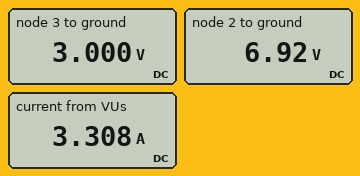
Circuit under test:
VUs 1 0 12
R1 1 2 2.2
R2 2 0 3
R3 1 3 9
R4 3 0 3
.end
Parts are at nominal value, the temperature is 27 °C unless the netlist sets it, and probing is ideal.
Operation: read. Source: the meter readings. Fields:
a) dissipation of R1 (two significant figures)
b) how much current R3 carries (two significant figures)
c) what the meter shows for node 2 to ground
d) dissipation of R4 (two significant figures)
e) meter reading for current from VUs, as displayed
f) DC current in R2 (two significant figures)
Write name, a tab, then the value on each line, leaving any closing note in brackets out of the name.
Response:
dissipation of R1	12 W
how much current R3 carries	1.0 A
what the meter shows for node 2 to ground	6.92 V
dissipation of R4	3.0 W
meter reading for current from VUs, as displayed	3.308 A
DC current in R2	2.3 A
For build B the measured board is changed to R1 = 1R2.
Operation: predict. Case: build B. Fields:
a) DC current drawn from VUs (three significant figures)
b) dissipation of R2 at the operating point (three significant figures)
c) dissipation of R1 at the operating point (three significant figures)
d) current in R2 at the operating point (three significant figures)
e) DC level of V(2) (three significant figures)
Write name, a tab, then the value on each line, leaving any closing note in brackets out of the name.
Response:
DC current drawn from VUs	3.86 A
dissipation of R2 at the operating point	24.5 W
dissipation of R1 at the operating point	9.80 W
current in R2 at the operating point	2.86 A
DC level of V(2)	8.57 V
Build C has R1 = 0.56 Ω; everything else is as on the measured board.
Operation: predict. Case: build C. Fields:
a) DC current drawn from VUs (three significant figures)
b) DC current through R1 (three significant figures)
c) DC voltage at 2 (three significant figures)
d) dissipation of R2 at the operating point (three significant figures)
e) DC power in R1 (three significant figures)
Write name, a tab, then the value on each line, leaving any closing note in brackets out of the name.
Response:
DC current drawn from VUs	4.37 A
DC current through R1	3.37 A
DC voltage at 2	10.1 V
dissipation of R2 at the operating point	34.1 W
DC power in R1	6.36 W
